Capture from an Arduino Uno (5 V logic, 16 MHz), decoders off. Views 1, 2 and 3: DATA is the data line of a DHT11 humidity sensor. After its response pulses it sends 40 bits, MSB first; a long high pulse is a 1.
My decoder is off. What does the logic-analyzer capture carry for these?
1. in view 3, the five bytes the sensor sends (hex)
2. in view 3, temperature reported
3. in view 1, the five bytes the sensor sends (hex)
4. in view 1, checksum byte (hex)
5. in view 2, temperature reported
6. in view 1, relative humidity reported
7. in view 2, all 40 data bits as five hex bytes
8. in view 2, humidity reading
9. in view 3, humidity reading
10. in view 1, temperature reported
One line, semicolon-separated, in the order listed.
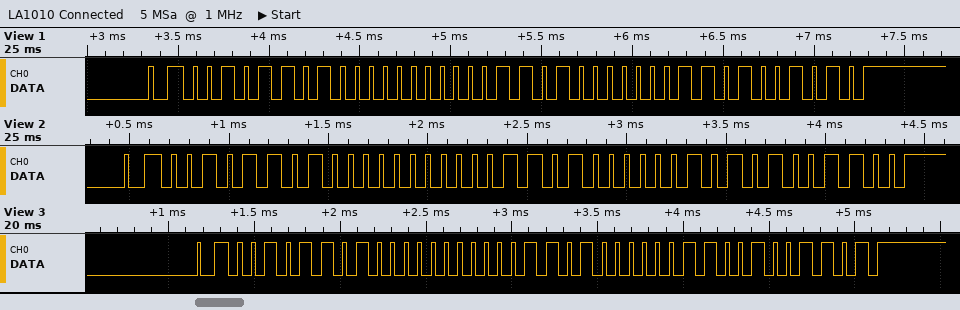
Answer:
2D 00 1A 06 4D; 26.6 °C; 2D 00 1A 03 4A; 0x4A; 26.5 °C; 45 %; 2D 00 1A 05 4C; 45 %; 45 %; 26.3 °C
